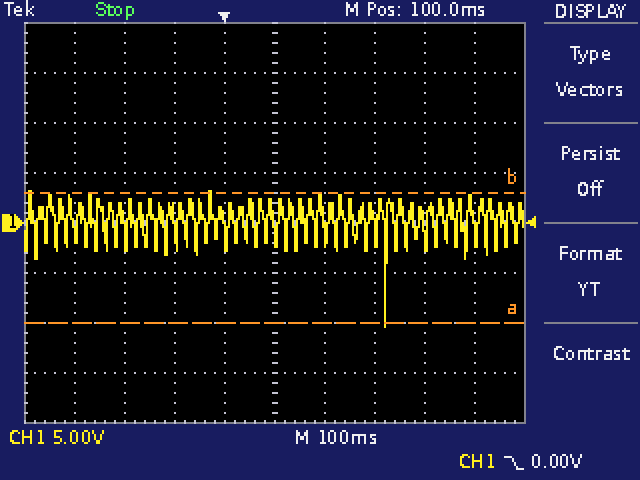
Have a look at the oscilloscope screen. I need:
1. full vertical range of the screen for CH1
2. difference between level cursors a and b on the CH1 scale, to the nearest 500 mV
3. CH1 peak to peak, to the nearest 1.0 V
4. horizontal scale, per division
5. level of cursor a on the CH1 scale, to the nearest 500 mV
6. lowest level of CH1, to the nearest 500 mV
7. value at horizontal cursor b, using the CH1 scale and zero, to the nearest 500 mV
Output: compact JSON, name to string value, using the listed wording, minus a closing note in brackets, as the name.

{"full vertical range of the screen for CH1": "40 V", "difference between level cursors a and b on the CH1 scale, to the nearest 500 mV": "13.0 V", "CH1 peak to peak, to the nearest 1.0 V": "14.0 V", "horizontal scale, per division": "100 ms", "level of cursor a on the CH1 scale, to the nearest 500 mV": "-10.0 V", "lowest level of CH1, to the nearest 500 mV": "-10.5 V", "value at horizontal cursor b, using the CH1 scale and zero, to the nearest 500 mV": "3.0 V"}
